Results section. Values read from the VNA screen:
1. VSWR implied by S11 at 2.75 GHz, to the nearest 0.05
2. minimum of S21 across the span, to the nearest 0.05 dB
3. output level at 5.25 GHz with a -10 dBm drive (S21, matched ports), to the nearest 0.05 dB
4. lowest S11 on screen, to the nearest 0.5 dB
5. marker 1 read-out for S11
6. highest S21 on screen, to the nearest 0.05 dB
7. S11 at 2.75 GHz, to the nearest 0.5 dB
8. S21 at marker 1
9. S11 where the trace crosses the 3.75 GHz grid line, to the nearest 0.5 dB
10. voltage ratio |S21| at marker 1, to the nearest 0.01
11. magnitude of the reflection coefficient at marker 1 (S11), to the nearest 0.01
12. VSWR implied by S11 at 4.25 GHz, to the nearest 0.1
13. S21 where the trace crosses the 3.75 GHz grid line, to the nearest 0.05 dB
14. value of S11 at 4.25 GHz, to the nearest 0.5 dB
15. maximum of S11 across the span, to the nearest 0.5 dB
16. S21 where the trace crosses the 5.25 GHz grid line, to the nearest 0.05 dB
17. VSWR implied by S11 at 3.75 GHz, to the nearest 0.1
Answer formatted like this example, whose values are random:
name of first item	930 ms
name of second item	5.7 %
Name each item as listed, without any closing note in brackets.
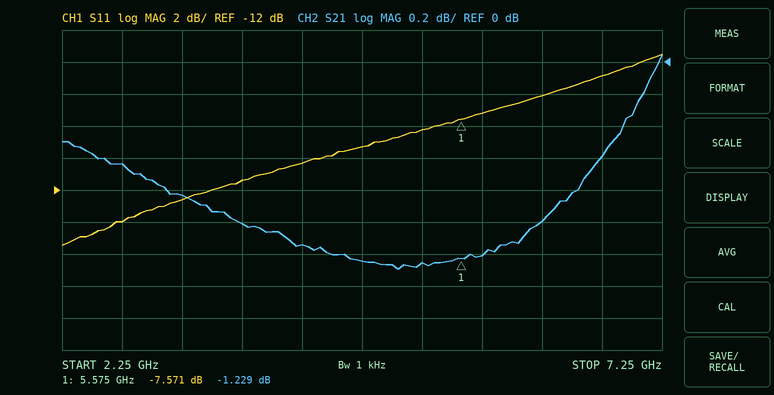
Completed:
VSWR implied by S11 at 2.75 GHz, to the nearest 0.05	1.50
minimum of S21 across the span, to the nearest 0.05 dB	-1.30 dB
output level at 5.25 GHz with a -10 dBm drive (S21, matched ports), to the nearest 0.05 dB	-11.25 dBm
lowest S11 on screen, to the nearest 0.5 dB	-15.5 dB
marker 1 read-out for S11	-7.571 dB
highest S21 on screen, to the nearest 0.05 dB	0.05 dB
S11 at 2.75 GHz, to the nearest 0.5 dB	-14.0 dB
S21 at marker 1	-1.229 dB
S11 where the trace crosses the 3.75 GHz grid line, to the nearest 0.5 dB	-11.5 dB
voltage ratio |S21| at marker 1, to the nearest 0.01	0.87
magnitude of the reflection coefficient at marker 1 (S11), to the nearest 0.01	0.42
VSWR implied by S11 at 4.25 GHz, to the nearest 0.1	1.9
S21 where the trace crosses the 3.75 GHz grid line, to the nearest 0.05 dB	-1.00 dB
value of S11 at 4.25 GHz, to the nearest 0.5 dB	-10.5 dB
maximum of S11 across the span, to the nearest 0.5 dB	-3.5 dB
S21 where the trace crosses the 5.25 GHz grid line, to the nearest 0.05 dB	-1.25 dB
VSWR implied by S11 at 3.75 GHz, to the nearest 0.1	1.7
